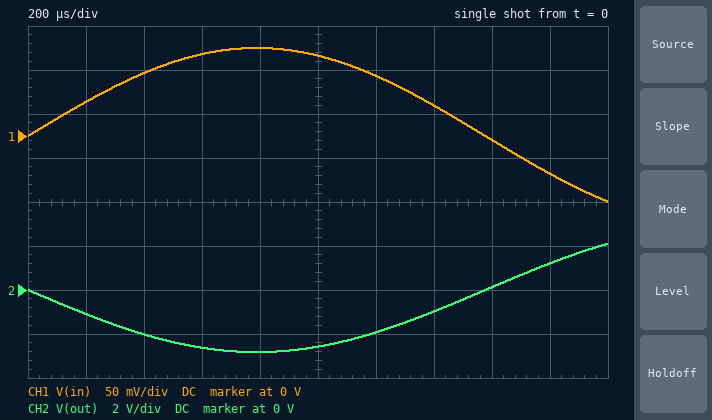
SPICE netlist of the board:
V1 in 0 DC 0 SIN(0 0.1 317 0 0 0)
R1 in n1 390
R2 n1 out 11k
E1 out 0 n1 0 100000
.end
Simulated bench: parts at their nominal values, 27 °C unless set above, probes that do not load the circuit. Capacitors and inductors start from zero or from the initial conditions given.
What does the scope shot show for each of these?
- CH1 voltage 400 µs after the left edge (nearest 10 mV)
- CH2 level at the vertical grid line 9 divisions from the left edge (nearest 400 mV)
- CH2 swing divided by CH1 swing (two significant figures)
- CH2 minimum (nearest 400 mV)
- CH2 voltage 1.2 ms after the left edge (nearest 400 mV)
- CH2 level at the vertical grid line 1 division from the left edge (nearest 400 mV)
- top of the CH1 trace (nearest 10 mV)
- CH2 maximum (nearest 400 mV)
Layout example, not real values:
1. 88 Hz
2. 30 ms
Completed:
1. 70 mV
2. 1.2 V
3. 28
4. -2.8 V
5. -2.0 V
6. -1.2 V
7. 100 mV
8. 2.0 V
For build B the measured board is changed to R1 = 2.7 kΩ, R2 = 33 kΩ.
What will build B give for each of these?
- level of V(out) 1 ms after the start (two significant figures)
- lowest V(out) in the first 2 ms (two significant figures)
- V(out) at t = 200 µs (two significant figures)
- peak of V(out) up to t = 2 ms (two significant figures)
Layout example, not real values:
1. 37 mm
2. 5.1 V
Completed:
1. -1.1 V
2. -1.2 V
3. -470 mV
4. 910 mV
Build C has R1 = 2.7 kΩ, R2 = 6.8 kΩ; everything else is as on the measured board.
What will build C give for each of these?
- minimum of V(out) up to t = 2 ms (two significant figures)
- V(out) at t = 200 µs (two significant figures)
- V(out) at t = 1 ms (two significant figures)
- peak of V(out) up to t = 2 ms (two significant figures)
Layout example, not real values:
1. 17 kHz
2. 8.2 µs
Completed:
1. -250 mV
2. -98 mV
3. -230 mV
4. 190 mV
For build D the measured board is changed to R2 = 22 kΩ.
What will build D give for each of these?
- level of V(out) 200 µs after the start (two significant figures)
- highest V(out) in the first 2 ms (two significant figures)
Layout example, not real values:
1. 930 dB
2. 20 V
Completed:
1. -2.2 V
2. 4.2 V
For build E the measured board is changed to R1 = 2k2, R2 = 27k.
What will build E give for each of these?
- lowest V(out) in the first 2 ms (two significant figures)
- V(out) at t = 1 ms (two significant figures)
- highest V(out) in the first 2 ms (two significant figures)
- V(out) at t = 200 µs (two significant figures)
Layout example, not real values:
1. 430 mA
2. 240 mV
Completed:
1. -1.2 V
2. -1.1 V
3. 920 mV
4. -480 mV
